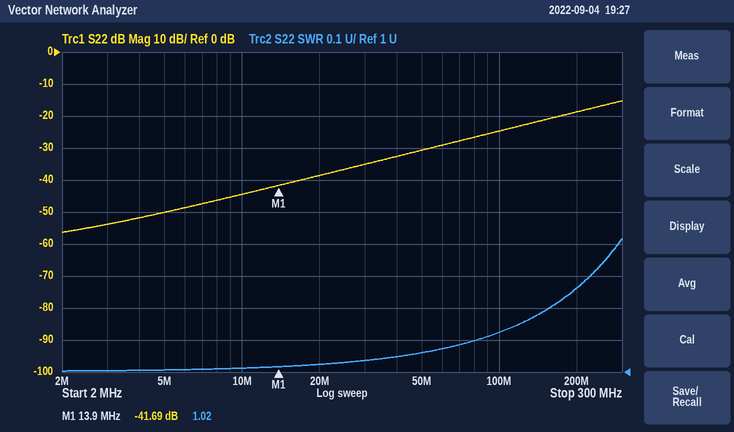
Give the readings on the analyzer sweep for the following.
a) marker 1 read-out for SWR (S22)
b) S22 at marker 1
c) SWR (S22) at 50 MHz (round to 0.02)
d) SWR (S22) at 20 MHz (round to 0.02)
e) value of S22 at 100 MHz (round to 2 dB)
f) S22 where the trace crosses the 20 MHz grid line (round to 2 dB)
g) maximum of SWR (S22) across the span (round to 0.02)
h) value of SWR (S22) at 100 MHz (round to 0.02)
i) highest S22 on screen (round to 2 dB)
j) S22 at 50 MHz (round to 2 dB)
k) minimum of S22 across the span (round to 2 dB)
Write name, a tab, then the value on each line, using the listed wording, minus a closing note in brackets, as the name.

marker 1 read-out for SWR	1.02
S22 at marker 1	-41.69 dB
SWR (S22) at 50 MHz	1.06
SWR (S22) at 20 MHz	1.02
value of S22 at 100 MHz	-24 dB
S22 where the trace crosses the 20 MHz grid line	-38 dB
maximum of SWR (S22) across the span	1.42
value of SWR (S22) at 100 MHz	1.12
highest S22 on screen	-16 dB
S22 at 50 MHz	-30 dB
minimum of S22 across the span	-56 dB
